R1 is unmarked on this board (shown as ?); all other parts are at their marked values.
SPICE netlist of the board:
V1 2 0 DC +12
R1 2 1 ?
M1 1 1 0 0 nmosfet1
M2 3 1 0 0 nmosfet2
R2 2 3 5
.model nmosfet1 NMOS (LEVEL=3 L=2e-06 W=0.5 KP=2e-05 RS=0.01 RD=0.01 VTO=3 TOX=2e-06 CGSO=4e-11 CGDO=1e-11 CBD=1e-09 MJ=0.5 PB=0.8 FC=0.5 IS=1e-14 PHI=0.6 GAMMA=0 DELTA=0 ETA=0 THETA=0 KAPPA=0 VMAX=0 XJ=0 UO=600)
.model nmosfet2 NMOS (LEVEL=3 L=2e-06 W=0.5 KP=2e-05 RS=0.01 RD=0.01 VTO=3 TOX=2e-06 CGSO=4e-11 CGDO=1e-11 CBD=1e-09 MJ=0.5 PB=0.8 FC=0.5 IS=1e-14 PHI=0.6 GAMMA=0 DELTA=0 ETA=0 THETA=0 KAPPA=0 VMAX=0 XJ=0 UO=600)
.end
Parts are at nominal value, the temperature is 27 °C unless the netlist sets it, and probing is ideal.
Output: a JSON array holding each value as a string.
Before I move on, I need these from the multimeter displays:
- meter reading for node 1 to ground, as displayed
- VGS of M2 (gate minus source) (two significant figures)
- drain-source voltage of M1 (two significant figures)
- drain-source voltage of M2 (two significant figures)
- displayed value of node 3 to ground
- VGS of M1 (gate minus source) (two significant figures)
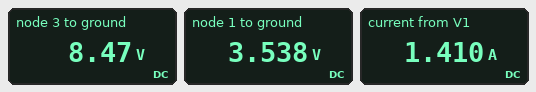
["3.538 V", "3.5 V", "3.5 V", "8.5 V", "8.47 V", "3.5 V"]
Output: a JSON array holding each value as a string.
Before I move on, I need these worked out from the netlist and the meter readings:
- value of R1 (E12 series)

["12 Ω"]
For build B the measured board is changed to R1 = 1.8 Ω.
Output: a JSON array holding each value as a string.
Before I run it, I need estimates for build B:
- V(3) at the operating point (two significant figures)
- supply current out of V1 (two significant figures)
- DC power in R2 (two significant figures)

["460 mV", "6.6 A", "27 W"]
